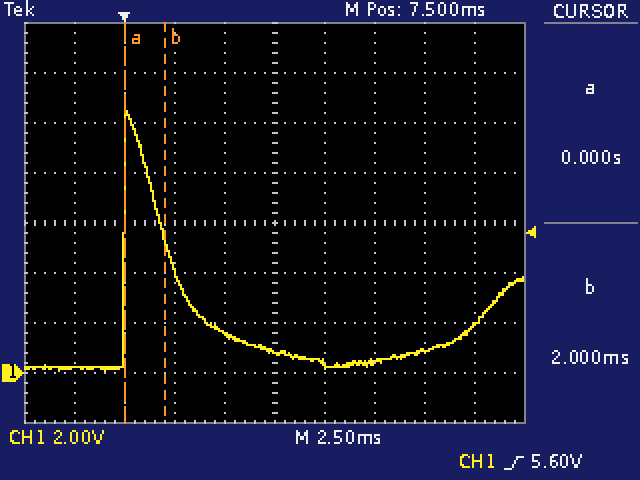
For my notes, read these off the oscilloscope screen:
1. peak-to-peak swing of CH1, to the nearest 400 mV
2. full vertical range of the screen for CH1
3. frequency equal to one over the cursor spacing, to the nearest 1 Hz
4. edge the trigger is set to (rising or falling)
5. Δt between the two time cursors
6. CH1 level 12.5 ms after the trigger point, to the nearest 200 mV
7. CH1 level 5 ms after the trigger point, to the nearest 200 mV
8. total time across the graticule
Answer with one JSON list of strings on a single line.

["10.4 V", "16 V", "500 Hz", "rising", "2.00 ms", "400 mV", "1.6 V", "25 ms"]
